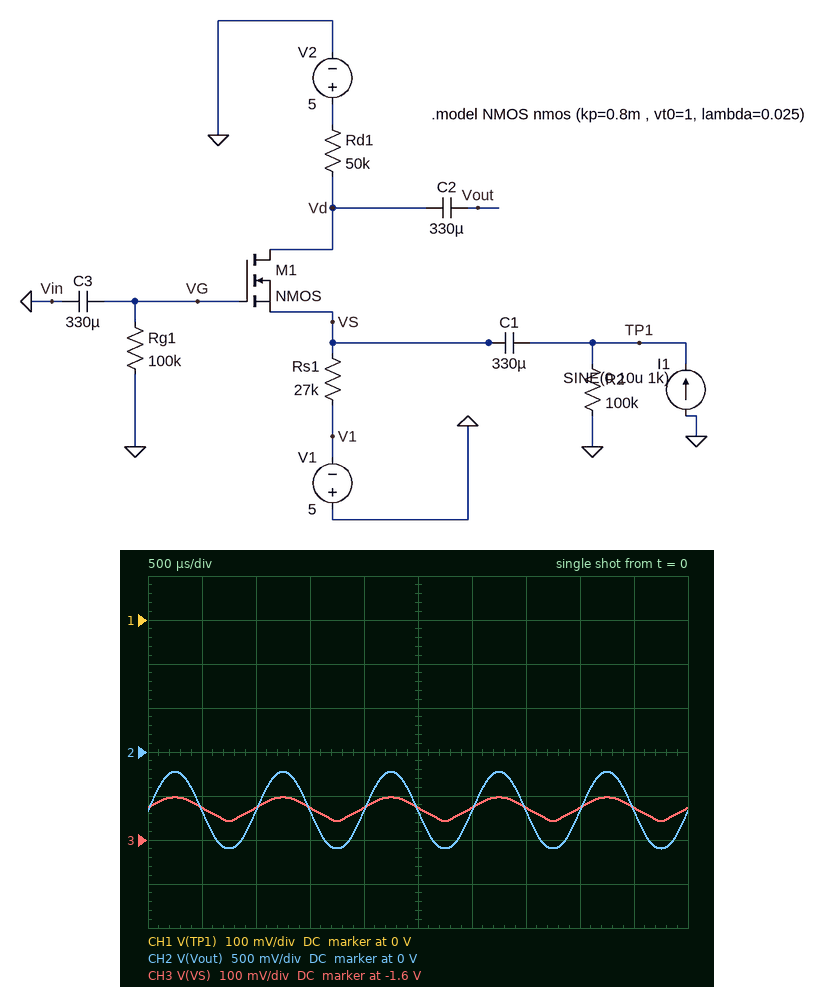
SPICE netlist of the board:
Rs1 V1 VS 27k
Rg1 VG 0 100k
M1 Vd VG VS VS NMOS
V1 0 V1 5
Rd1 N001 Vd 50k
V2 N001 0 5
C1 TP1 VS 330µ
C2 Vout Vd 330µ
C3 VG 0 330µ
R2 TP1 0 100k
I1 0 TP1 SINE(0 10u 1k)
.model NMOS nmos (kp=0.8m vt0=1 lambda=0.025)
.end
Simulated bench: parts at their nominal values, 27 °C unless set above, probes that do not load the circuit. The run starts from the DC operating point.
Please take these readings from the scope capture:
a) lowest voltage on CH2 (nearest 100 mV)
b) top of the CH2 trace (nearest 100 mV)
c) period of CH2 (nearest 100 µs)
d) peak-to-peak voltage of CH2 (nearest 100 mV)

-1.1 V
-200 mV
1.0 ms
900 mV
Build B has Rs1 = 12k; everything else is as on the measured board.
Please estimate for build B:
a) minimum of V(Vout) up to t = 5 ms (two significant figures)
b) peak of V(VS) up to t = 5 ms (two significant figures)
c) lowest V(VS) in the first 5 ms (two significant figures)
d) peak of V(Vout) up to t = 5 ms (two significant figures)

-2.8 V
-2.7 V
-2.9 V
-2.6 V
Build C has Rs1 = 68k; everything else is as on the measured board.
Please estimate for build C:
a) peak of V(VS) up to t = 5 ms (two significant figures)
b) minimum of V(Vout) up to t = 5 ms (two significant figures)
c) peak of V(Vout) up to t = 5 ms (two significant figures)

-1.3 V
2.5 V
3.4 V
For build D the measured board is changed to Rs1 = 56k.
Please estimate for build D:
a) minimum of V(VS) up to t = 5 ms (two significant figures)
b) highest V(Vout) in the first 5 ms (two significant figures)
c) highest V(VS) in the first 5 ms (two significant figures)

-1.4 V
2.9 V
-1.3 V
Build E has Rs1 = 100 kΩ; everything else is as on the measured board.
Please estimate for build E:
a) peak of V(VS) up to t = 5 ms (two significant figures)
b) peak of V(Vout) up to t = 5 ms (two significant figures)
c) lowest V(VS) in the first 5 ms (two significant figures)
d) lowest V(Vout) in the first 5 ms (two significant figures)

-1.2 V
4.2 V
-1.3 V
3.3 V
